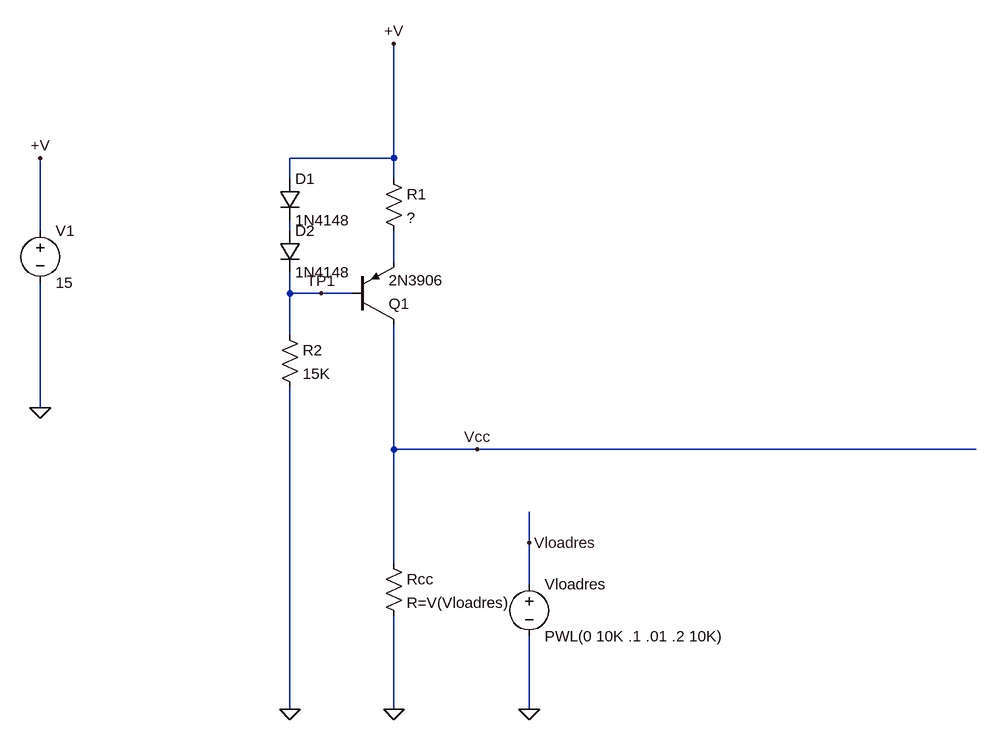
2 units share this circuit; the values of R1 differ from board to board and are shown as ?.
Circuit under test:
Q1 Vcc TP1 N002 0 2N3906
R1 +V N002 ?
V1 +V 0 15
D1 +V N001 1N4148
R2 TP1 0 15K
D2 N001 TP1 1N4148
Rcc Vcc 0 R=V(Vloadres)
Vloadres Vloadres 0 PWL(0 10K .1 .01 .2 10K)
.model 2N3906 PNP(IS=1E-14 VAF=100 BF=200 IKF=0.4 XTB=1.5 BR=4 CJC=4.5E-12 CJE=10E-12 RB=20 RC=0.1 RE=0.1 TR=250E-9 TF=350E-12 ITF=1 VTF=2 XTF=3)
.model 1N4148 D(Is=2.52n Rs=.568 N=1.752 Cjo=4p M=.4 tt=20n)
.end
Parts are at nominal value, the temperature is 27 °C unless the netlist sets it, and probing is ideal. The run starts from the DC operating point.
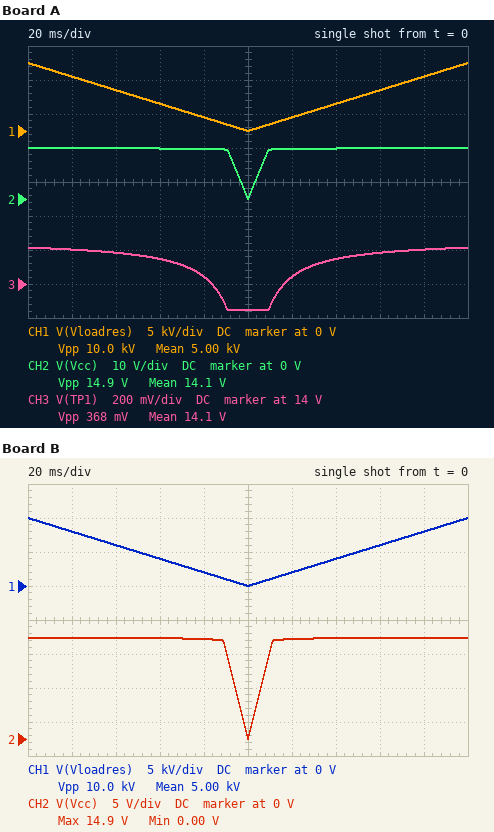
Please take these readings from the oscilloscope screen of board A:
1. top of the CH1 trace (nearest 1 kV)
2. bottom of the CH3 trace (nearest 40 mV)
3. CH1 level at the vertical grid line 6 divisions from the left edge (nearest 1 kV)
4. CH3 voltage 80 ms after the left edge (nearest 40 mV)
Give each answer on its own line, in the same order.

10 kV
13.84 V
2 kV
14.04 V
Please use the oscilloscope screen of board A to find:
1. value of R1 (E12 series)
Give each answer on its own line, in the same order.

27 Ω
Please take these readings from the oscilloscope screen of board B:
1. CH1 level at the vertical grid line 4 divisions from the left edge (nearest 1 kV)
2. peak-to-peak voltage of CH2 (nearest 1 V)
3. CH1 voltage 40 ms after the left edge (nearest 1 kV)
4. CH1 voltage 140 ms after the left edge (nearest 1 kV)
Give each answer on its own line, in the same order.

2 kV
15 V
6 kV
4 kV
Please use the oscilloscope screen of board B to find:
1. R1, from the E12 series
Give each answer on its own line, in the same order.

33 Ω
